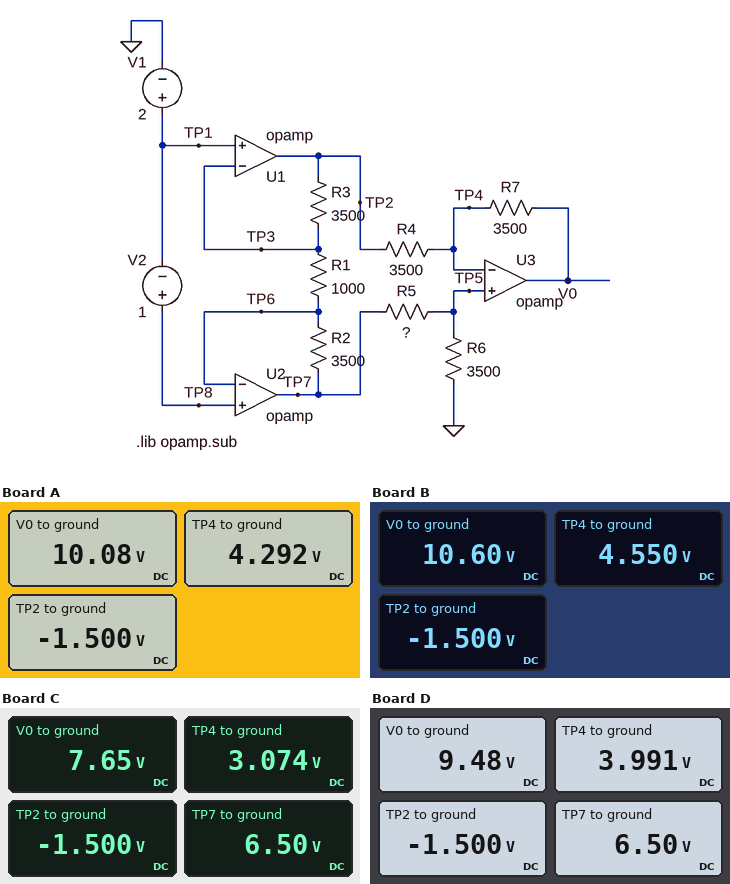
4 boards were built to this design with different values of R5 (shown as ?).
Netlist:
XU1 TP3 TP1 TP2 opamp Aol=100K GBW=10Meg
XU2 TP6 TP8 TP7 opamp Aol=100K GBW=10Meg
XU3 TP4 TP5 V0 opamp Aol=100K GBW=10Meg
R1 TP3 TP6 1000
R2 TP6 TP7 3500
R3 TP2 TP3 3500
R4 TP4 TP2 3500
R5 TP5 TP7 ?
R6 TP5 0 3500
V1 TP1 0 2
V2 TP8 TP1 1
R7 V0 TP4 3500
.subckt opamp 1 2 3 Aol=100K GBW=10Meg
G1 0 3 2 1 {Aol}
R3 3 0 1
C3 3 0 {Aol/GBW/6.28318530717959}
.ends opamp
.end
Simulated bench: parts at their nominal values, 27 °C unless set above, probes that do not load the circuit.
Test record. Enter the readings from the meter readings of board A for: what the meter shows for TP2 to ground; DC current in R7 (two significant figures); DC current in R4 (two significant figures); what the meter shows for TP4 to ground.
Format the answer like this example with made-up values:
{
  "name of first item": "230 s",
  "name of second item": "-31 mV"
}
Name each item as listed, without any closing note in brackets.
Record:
{
  "what the meter shows for TP2 to ground": "-1.500 V",
  "DC current in R7": "1.7 mA",
  "DC current in R4": "1.7 mA",
  "what the meter shows for TP4 to ground": "4.292 V"
}
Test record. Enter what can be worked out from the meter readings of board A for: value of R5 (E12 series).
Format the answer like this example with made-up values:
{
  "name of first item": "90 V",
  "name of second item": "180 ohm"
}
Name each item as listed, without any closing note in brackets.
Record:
{
  "value of R5": "1.8 kΩ"
}
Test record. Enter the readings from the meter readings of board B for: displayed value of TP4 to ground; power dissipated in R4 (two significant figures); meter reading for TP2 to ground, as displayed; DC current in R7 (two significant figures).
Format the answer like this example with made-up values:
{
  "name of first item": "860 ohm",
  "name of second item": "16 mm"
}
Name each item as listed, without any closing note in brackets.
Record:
{
  "displayed value of TP4 to ground": "4.550 V",
  "power dissipated in R4": "10 mW",
  "meter reading for TP2 to ground, as displayed": "-1.500 V",
  "DC current in R7": "1.7 mA"
}
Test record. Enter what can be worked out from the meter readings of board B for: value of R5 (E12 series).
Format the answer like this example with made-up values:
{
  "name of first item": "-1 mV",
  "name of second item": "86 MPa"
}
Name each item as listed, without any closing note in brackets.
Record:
{
  "value of R5": "1.5 kΩ"
}
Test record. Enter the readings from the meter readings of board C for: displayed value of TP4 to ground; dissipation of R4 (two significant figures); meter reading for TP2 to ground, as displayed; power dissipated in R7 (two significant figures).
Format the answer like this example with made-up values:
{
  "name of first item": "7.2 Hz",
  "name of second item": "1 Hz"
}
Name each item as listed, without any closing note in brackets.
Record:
{
  "displayed value of TP4 to ground": "3.074 V",
  "dissipation of R4": "6.0 mW",
  "meter reading for TP2 to ground, as displayed": "-1.500 V",
  "power dissipated in R7": "6.0 mW"
}
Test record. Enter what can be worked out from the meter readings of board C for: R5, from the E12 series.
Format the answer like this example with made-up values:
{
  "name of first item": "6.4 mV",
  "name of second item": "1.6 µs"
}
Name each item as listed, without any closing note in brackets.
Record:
{
  "R5, from the E12 series": "3.9 kΩ"
}
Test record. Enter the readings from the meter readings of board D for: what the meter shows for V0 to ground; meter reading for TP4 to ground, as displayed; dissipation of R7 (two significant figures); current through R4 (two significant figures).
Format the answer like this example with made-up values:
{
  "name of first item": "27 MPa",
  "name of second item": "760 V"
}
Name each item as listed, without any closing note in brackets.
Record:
{
  "what the meter shows for V0 to ground": "9.48 V",
  "meter reading for TP4 to ground, as displayed": "3.991 V",
  "dissipation of R7": "8.6 mW",
  "current through R4": "1.6 mA"
}
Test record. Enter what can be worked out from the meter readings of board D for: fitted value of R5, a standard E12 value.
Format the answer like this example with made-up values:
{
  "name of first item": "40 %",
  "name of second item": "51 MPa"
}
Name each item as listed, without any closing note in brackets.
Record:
{
  "fitted value of R5, a standard E12 value": "2.2 kΩ"
}
